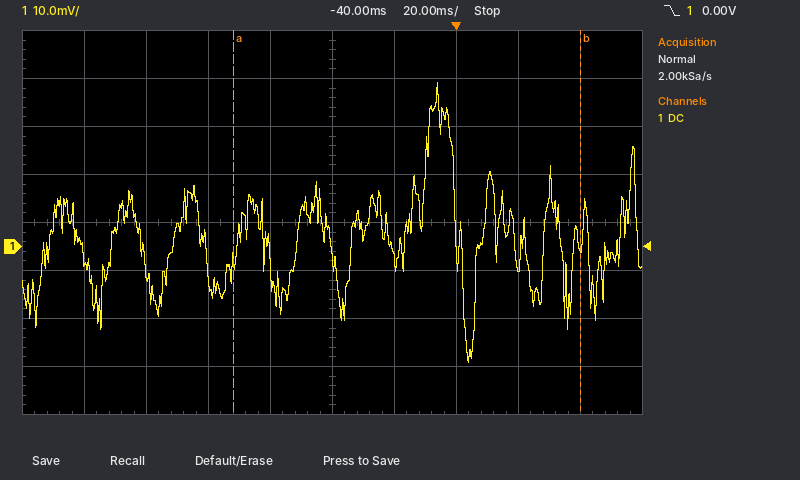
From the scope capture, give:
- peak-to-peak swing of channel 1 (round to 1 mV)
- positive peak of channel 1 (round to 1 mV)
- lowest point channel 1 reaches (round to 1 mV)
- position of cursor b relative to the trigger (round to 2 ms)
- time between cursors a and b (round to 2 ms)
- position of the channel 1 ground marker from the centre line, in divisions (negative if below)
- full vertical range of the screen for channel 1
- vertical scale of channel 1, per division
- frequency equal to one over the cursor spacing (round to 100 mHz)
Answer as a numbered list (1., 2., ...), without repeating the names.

1. 58 mV
2. 34 mV
3. -24 mV
4. +40 ms
5. 112 ms
6. -0.5 div
7. 80 mV
8. 10 mV
9. 8.9 Hz
